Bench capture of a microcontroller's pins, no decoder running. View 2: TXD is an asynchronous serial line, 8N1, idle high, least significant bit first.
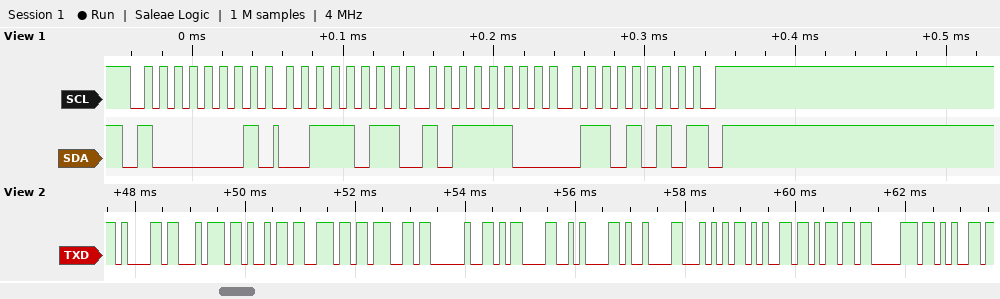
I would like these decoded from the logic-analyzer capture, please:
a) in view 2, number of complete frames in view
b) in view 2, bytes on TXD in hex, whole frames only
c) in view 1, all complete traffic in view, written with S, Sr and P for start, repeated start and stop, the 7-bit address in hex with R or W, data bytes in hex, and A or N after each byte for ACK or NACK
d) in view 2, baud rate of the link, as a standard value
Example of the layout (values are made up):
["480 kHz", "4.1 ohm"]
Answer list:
["14", "0x61 0x74 0x69 0x6E 0x67 0x20 0x0D 0x0A 0x09 0x54 0x65 0x6D 0x70 0x65", "S 40R A 3B A BC A 6A N P", "9600 baud"]
